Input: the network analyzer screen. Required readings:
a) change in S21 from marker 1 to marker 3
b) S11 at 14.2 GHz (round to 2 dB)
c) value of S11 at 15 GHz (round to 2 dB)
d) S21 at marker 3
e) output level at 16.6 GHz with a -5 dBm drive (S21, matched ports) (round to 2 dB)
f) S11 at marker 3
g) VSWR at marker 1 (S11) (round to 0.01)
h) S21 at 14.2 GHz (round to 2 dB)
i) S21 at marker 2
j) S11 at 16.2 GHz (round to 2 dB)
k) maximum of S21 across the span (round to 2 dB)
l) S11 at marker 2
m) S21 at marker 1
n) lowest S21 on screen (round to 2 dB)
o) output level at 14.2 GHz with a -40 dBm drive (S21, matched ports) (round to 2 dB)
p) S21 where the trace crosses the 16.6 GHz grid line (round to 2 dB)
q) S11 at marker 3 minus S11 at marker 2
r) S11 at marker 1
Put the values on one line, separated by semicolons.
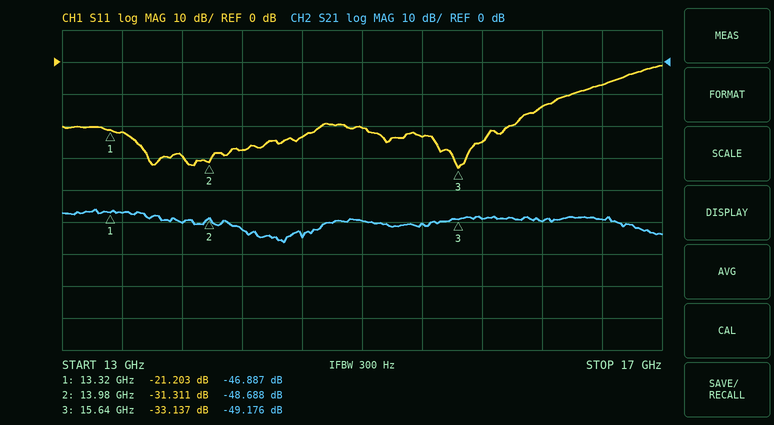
-2.289 dB; -28 dB; -20 dB; -49.176 dB; -54 dBm; -33.137 dB; 1.19; -52 dB; -48.688 dB; -14 dB; -46 dB; -31.311 dB; -46.887 dB; -56 dB; -92 dBm; -50 dB; -1.826 dB; -21.203 dB
